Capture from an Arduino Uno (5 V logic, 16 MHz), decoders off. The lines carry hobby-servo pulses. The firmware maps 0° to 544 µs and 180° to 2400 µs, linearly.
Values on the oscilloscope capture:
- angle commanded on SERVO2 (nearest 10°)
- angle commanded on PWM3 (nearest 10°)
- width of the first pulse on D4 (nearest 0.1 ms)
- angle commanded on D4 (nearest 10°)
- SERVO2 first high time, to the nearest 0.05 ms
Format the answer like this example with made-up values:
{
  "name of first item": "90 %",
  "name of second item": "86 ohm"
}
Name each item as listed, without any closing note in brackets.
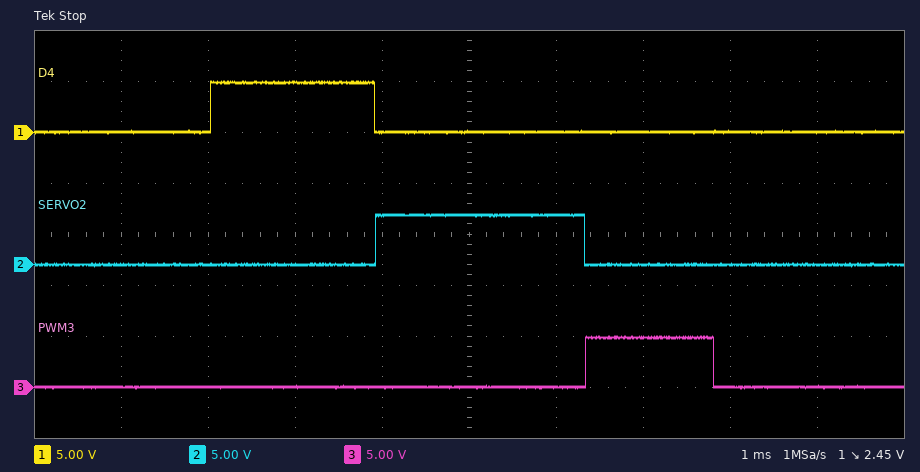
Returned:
{
  "angle commanded on SERVO2": "180°",
  "angle commanded on PWM3": "90°",
  "width of the first pulse on D4": "1.9 ms",
  "angle commanded on D4": "130°",
  "SERVO2 first high time, to the nearest 0.05 ms": "2.40 ms"
}
